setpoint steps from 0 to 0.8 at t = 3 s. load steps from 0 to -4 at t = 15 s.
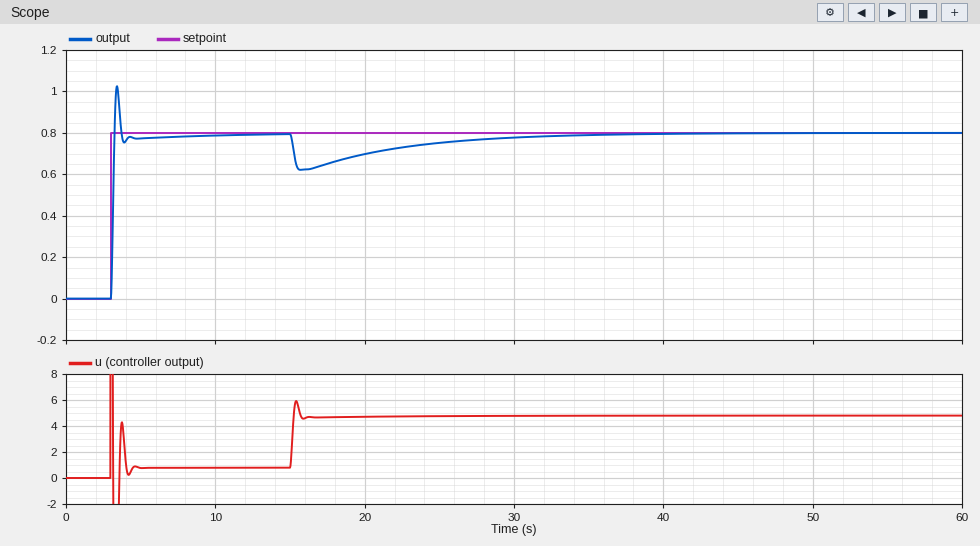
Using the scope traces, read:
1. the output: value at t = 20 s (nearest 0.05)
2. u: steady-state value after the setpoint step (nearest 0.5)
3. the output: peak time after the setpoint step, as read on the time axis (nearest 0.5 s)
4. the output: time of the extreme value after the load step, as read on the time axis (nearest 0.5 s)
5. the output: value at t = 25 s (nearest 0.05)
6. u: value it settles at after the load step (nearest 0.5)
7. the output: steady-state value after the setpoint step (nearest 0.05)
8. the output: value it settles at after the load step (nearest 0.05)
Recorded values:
0.70
1.0
3.5 s
15.5 s
0.75
5.0
0.80
0.80
